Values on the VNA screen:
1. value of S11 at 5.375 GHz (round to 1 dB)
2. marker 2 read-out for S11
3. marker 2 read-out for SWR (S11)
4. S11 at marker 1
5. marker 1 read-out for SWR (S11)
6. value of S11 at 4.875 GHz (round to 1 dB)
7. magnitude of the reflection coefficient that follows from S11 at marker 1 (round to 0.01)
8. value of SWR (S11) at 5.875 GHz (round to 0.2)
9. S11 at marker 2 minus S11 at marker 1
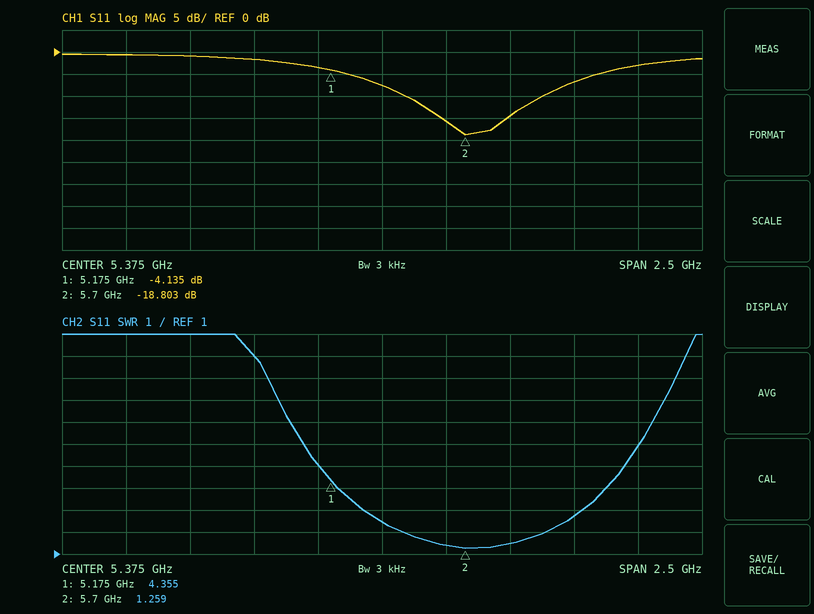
-8 dB
-18.803 dB
1.259
-4.135 dB
4.355
-2 dB
0.62
1.4
-14.668 dB
